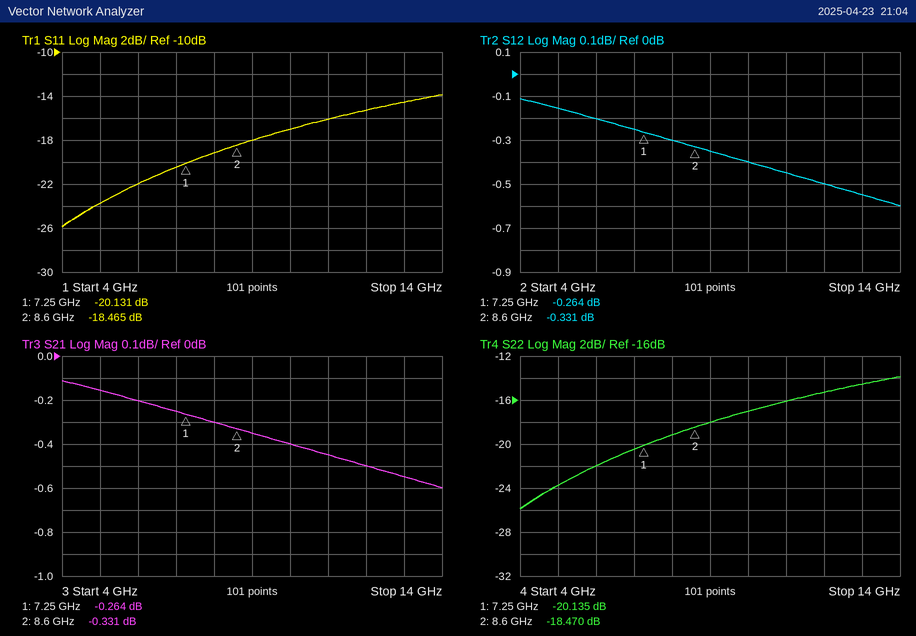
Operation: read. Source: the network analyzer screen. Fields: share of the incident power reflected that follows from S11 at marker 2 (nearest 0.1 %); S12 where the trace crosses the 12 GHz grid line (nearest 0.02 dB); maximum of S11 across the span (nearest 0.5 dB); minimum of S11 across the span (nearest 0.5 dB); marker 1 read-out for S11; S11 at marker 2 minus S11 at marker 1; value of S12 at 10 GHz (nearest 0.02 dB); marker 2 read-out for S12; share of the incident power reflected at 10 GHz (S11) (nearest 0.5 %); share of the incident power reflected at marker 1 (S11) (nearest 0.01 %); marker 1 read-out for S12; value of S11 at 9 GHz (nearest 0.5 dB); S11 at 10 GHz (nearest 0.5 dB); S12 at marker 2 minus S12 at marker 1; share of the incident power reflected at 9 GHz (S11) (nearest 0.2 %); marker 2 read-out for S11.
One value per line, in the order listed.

1.4 %
-0.50 dB
-14.0 dB
-26.0 dB
-20.131 dB
1.666 dB
-0.40 dB
-0.331 dB
2.0 %
0.97 %
-0.264 dB
-18.0 dB
-17.0 dB
-0.067 dB
1.6 %
-18.465 dB
